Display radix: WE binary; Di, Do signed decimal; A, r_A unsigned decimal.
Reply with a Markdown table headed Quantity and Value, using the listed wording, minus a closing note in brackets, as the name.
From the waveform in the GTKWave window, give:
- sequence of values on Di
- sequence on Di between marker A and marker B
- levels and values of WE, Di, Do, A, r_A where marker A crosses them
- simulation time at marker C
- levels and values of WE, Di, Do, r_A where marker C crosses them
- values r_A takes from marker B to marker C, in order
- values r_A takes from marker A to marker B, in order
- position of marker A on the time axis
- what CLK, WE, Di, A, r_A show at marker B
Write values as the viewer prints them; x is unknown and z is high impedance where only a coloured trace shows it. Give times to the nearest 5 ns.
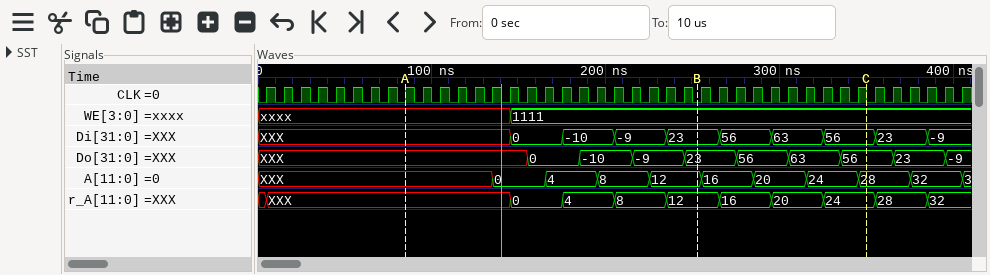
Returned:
| Quantity | Value |
|---|---|
| sequence of values on Di | XXX, 0, -10, -9, 23, 56, 63, 56, 23, -9 |
| sequence on Di between marker A and marker B | XXX, 0, -10, -9, 23 |
| levels and values of WE, Di, Do, A, r_A where marker A crosses them | WE=xxxx, Di=XXX, Do=XXX, A=XXX, r_A=XXX |
| simulation time at marker C | 350 ns |
| levels and values of WE, Di, Do, r_A where marker C crosses them | WE=1111, Di=56, Do=56, r_A=24 |
| values r_A takes from marker B to marker C, in order | 12, 16, 20, 24 |
| values r_A takes from marker A to marker B, in order | XXX, 0, 4, 8, 12 |
| position of marker A on the time axis | 85 ns |
| what CLK, WE, Di, A, r_A show at marker B | CLK=0, WE=1111, Di=23, A=12, r_A=12 |
